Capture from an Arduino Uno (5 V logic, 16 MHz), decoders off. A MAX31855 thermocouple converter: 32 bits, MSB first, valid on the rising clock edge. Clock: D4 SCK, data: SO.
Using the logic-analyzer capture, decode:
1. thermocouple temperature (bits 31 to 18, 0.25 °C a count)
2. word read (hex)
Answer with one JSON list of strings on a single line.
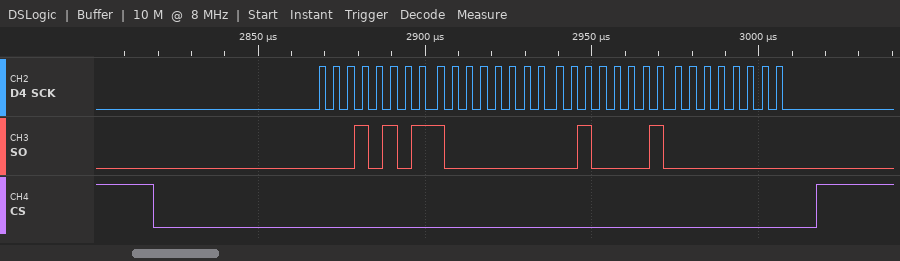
["344.00 °C", "0x15802100"]
